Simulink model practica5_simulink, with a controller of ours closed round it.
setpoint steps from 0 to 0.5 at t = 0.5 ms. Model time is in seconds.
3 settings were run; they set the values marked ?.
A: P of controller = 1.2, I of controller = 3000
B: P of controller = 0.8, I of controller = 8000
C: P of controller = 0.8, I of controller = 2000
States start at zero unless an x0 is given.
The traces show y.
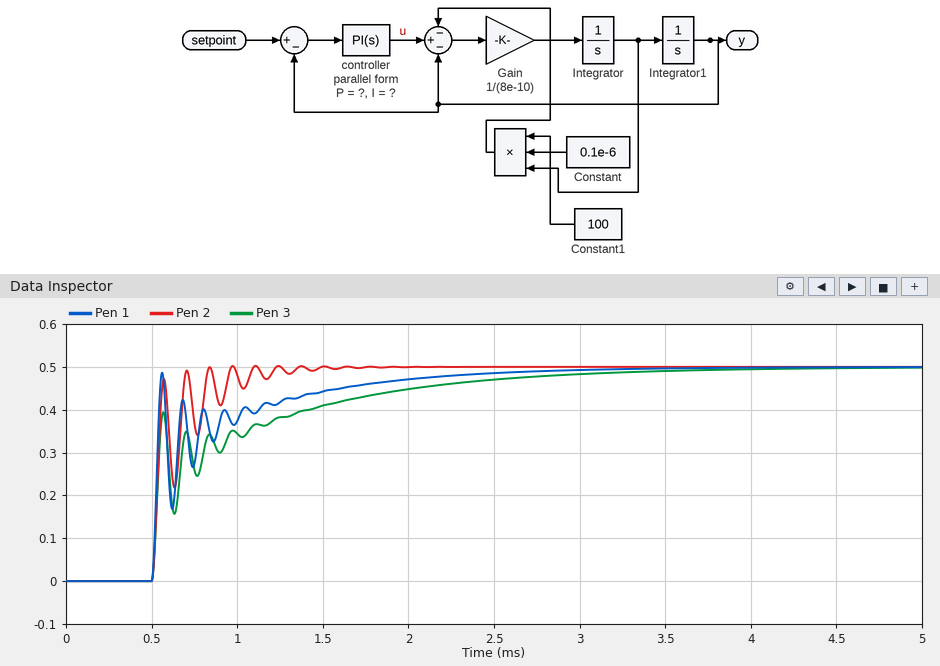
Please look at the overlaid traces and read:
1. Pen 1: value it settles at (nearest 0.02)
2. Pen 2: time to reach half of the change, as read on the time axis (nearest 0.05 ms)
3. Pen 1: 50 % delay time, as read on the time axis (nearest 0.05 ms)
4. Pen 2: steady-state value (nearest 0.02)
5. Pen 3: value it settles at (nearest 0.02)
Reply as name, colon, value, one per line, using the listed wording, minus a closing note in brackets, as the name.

Pen 1: value it settles at: 0.50
Pen 2: time to reach half of the change, as read on the time axis: 0.55 ms
Pen 1: 50 % delay time, as read on the time axis: 0.55 ms
Pen 2: steady-state value: 0.50
Pen 3: value it settles at: 0.50
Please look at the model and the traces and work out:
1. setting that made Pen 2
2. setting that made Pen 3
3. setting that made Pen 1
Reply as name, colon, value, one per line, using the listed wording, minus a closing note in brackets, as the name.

setting that made Pen 2: B
setting that made Pen 3: C
setting that made Pen 1: A
